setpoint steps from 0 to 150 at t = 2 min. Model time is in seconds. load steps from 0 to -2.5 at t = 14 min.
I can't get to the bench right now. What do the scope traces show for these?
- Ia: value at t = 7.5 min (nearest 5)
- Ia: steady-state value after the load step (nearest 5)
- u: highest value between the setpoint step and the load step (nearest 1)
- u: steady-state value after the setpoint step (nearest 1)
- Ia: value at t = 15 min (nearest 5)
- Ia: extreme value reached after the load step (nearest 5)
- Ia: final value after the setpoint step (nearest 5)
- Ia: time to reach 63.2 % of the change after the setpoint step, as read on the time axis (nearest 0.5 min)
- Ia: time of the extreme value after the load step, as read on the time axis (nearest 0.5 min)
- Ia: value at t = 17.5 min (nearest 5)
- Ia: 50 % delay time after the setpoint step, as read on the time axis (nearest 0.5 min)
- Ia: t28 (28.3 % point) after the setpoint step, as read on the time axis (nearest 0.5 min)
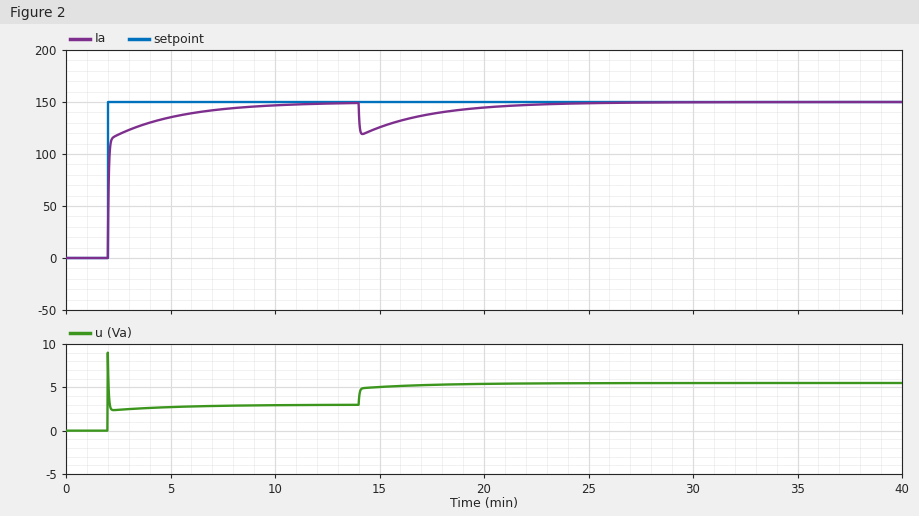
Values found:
145
150
9
3
125
120
150
2.0 min
14.0 min
140
2.0 min
2.0 min
